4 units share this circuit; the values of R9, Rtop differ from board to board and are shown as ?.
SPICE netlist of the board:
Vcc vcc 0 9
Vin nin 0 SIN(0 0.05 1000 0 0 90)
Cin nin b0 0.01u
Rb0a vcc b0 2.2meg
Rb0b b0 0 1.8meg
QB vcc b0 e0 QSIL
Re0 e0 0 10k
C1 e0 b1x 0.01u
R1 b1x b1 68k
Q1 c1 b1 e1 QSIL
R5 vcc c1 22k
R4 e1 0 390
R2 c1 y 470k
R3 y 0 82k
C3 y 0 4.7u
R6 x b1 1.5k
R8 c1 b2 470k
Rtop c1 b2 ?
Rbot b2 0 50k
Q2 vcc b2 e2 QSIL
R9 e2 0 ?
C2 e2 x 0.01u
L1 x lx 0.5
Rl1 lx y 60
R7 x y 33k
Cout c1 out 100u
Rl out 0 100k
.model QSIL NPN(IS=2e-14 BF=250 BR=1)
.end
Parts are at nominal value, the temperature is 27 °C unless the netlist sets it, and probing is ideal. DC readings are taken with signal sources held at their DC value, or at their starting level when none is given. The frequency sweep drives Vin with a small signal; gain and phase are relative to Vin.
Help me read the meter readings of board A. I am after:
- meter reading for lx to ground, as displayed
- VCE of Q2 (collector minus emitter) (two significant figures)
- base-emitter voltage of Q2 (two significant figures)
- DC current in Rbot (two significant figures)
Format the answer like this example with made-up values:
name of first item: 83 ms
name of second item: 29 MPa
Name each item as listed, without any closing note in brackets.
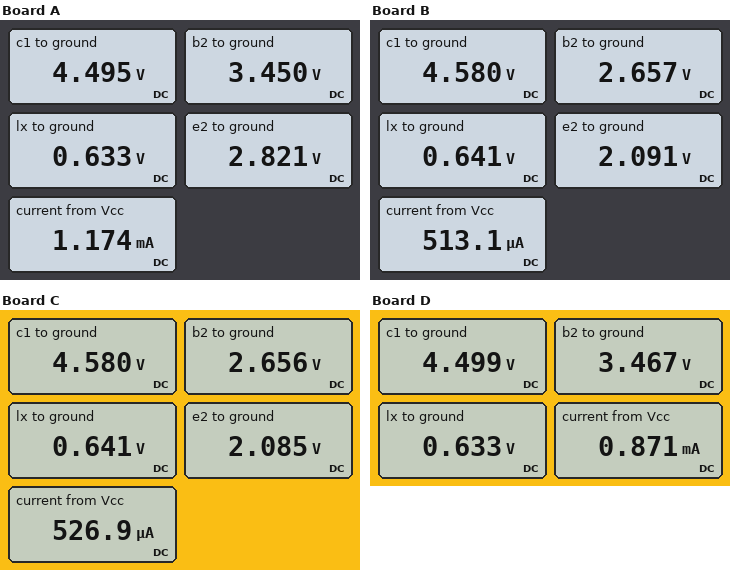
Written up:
meter reading for lx to ground, as displayed: 0.633 V
VCE of Q2 (collector minus emitter): 6.2 V
base-emitter voltage of Q2: 630 mV
DC current in Rbot: 69 µA
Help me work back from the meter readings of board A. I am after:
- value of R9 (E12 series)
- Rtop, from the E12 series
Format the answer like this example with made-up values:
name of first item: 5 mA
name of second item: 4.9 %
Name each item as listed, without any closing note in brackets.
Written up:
value of R9: 3.9 kΩ
Rtop, from the E12 series: 15 kΩ
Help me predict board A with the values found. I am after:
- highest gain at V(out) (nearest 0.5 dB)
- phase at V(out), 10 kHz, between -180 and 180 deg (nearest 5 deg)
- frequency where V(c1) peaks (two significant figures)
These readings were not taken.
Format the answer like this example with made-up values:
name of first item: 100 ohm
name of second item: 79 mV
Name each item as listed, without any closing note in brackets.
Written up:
highest gain at V(out): 14.5 dB
phase at V(out), 10 kHz, between -180 and 180 deg: 135 deg
frequency where V(c1) peaks: 540 Hz
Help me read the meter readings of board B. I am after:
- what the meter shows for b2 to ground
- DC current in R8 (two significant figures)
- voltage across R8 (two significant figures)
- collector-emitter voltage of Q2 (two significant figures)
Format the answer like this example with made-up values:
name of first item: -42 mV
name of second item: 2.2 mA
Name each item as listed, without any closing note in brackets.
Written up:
what the meter shows for b2 to ground: 2.657 V
DC current in R8: 4.1 µA
voltage across R8: 1.9 V
collector-emitter voltage of Q2: 6.9 V
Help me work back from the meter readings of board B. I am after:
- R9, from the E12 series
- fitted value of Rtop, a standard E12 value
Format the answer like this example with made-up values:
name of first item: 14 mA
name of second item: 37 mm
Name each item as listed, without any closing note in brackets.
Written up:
R9, from the E12 series: 33 kΩ
fitted value of Rtop, a standard E12 value: 39 kΩ
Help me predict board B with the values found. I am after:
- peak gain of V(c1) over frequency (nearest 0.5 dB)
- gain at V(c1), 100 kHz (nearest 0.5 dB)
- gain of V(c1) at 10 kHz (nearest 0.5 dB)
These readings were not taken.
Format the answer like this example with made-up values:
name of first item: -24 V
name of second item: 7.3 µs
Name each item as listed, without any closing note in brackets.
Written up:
peak gain of V(c1) over frequency: 14.5 dB
gain at V(c1), 100 kHz: -26.5 dB
gain of V(c1) at 10 kHz: -24.5 dB
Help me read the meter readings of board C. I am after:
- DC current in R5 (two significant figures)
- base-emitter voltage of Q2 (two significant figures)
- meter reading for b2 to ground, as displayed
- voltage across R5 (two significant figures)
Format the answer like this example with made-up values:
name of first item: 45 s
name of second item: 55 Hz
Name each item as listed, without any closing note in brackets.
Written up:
DC current in R5: 200 µA
base-emitter voltage of Q2: 570 mV
meter reading for b2 to ground, as displayed: 2.656 V
voltage across R5: 4.4 V
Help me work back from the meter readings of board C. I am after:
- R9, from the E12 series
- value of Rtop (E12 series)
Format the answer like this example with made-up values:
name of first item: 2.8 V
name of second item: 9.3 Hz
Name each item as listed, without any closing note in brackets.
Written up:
R9, from the E12 series: 27 kΩ
value of Rtop: 39 kΩ
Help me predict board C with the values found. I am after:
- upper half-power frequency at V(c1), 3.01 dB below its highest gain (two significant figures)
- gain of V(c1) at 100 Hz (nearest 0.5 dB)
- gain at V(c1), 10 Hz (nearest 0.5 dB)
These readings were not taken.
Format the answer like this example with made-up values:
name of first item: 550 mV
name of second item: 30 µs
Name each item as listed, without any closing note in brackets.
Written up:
upper half-power frequency at V(c1), 3.01 dB below its highest gain: 630 Hz
gain of V(c1) at 100 Hz: -13.5 dB
gain at V(c1), 10 Hz: -33.0 dB
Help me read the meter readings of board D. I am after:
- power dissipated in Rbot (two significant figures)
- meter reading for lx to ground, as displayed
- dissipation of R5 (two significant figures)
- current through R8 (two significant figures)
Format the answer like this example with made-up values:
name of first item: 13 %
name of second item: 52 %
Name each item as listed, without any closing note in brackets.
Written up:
power dissipated in Rbot: 240 µW
meter reading for lx to ground, as displayed: 0.633 V
dissipation of R5: 920 µW
current through R8: 2.2 µA
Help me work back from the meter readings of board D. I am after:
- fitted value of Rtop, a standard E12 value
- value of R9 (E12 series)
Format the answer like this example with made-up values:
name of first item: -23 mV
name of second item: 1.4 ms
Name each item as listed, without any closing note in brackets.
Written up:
fitted value of Rtop, a standard E12 value: 15 kΩ
value of R9: 6.8 kΩ
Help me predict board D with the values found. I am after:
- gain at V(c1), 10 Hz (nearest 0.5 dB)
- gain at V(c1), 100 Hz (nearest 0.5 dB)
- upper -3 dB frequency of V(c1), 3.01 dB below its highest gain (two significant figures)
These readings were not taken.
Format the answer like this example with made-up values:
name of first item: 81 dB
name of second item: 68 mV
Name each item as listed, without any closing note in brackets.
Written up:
gain at V(c1), 10 Hz: -34.0 dB
gain at V(c1), 100 Hz: -14.0 dB
upper -3 dB frequency of V(c1), 3.01 dB below its highest gain: 570 Hz
